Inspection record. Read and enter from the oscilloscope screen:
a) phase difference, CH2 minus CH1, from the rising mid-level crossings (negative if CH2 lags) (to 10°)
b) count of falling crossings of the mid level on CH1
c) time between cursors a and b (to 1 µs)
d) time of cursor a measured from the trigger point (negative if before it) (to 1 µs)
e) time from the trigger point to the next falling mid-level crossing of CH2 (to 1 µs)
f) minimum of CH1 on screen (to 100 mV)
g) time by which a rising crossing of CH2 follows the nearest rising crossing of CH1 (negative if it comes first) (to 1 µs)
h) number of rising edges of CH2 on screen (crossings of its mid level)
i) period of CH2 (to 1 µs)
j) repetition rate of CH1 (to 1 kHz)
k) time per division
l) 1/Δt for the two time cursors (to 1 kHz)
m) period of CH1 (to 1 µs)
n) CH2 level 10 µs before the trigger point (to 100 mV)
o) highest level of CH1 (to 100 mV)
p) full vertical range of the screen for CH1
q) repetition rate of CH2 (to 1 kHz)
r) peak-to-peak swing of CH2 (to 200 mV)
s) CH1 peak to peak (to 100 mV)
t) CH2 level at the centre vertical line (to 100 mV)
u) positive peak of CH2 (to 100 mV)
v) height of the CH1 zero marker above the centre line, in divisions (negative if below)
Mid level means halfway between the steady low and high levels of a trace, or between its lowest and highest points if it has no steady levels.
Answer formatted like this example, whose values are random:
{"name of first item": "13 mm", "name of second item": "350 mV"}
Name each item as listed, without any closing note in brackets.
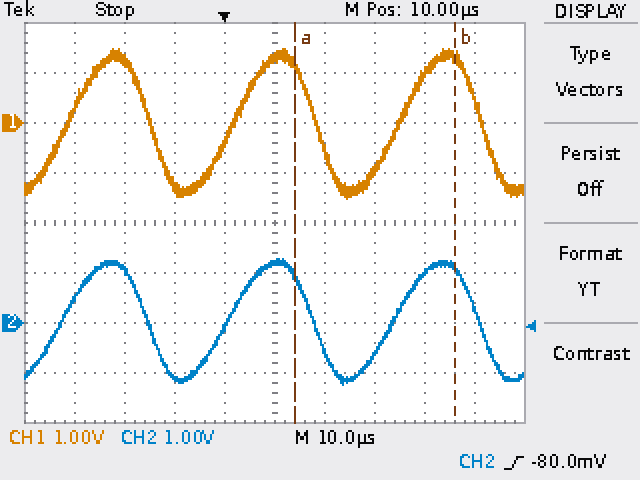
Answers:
{"phase difference, CH2 minus CH1, from the rising mid-level crossings (negative if CH2 lags)": "+10°", "count of falling crossings of the mid level on CH1": "3", "time between cursors a and b": "32 µs", "time of cursor a measured from the trigger point (negative if before it)": "+14 µs", "time from the trigger point to the next falling mid-level crossing of CH2": "18 µs", "minimum of CH1 on screen": "-1.5 V", "time by which a rising crossing of CH2 follows the nearest rising crossing of CH1 (negative if it comes first)": "-1 µs", "number of rising edges of CH2 on screen": "3", "period of CH2": "33 µs", "repetition rate of CH1": "30 kHz", "time per division": "10 µs", "1/Δt for the two time cursors": "31 kHz", "period of CH1": "33 µs", "CH2 level 10 µs before the trigger point": "-1.1 V", "highest level of CH1": "1.5 V", "full vertical range of the screen for CH1": "8 V", "repetition rate of CH2": "30 kHz", "peak-to-peak swing of CH2": "2.6 V", "CH1 peak to peak": "3.0 V", "CH2 level at the centre vertical line": "1.2 V", "positive peak of CH2": "1.3 V", "height of the CH1 zero marker above the centre line, in divisions": "+2.0 div"}
